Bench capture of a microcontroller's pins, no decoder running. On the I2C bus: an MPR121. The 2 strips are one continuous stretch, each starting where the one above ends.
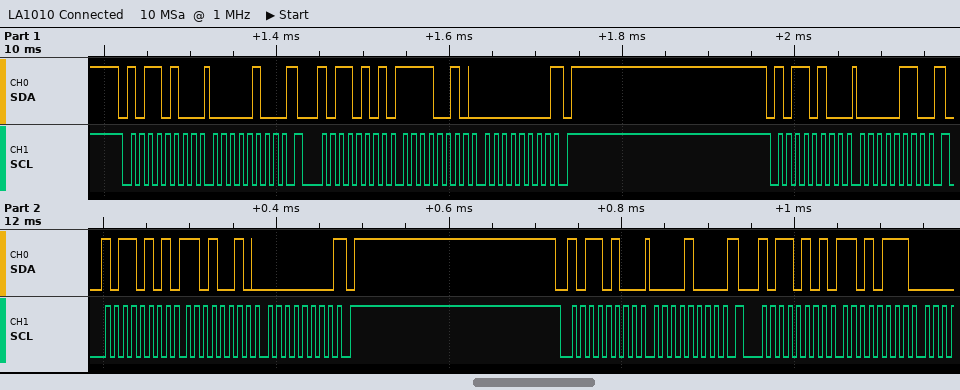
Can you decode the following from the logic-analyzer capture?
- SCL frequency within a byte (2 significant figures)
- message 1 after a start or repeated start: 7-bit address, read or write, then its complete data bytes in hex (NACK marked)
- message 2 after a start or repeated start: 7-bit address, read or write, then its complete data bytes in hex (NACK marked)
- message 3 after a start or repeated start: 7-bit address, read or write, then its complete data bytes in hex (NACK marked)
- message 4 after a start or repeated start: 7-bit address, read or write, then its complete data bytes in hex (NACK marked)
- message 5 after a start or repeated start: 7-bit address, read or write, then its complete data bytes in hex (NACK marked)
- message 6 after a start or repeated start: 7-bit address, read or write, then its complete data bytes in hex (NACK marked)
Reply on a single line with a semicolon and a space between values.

100 kHz; 0x5A write: 04; 0x5A read: F2 00 NACK; 0x5A write: 06; 0x5A read: D2 00 NACK; 0x5A write: 08; 0x5A read: D7
